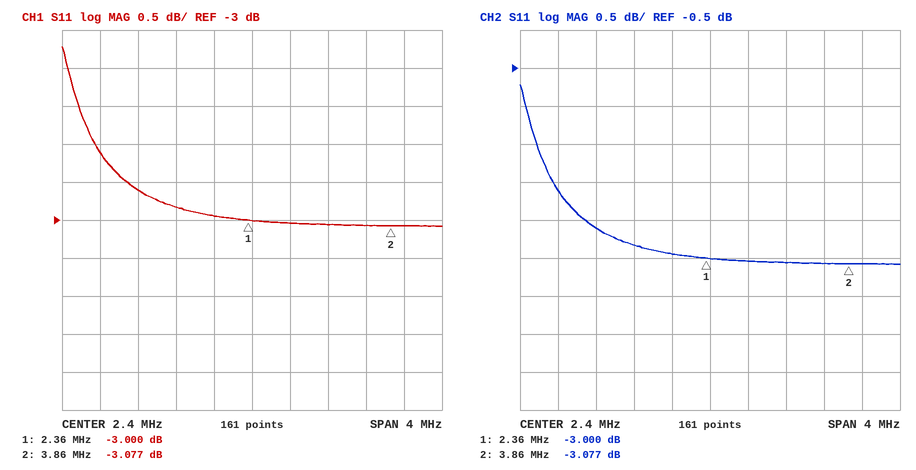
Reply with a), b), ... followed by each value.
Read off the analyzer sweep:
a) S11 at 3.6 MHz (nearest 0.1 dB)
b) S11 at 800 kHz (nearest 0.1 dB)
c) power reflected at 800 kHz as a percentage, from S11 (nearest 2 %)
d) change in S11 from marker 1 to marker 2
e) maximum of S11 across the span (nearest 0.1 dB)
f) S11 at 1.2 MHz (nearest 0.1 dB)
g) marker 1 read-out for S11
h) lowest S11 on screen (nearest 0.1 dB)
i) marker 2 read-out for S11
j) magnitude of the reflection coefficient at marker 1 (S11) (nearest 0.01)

a) -3.1 dB
b) -2.1 dB
c) 62 %
d) -0.077 dB
e) -0.7 dB
f) -2.6 dB
g) -3.000 dB
h) -3.1 dB
i) -3.077 dB
j) 0.71
